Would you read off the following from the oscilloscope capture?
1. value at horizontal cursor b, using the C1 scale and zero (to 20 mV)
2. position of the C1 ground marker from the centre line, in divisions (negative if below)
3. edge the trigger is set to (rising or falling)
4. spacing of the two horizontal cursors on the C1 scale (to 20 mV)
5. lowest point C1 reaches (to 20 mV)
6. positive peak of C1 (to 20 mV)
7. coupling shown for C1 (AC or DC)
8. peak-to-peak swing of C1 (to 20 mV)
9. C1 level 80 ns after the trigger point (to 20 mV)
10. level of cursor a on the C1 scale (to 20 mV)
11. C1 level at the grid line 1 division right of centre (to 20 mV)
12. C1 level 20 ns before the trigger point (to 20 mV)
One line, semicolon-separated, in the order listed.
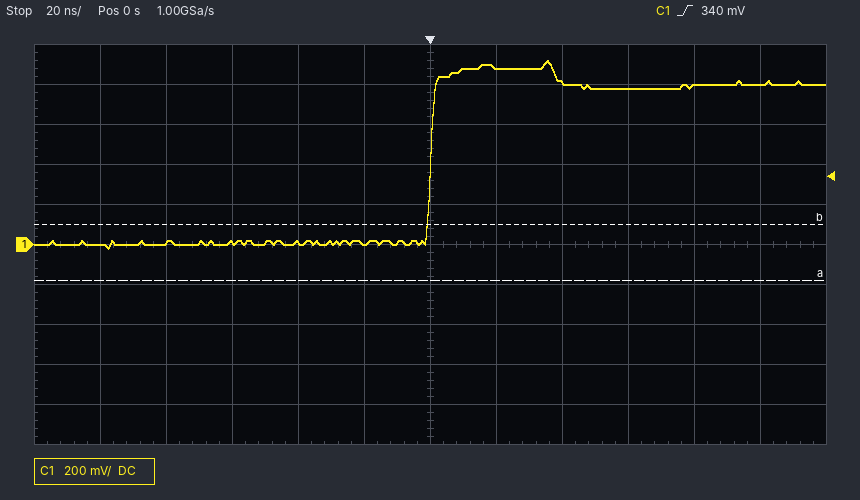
100 mV; 0.0 div; rising; 280 mV; -20 mV; 920 mV; DC; 940 mV; 800 mV; -180 mV; 880 mV; 0 mV
